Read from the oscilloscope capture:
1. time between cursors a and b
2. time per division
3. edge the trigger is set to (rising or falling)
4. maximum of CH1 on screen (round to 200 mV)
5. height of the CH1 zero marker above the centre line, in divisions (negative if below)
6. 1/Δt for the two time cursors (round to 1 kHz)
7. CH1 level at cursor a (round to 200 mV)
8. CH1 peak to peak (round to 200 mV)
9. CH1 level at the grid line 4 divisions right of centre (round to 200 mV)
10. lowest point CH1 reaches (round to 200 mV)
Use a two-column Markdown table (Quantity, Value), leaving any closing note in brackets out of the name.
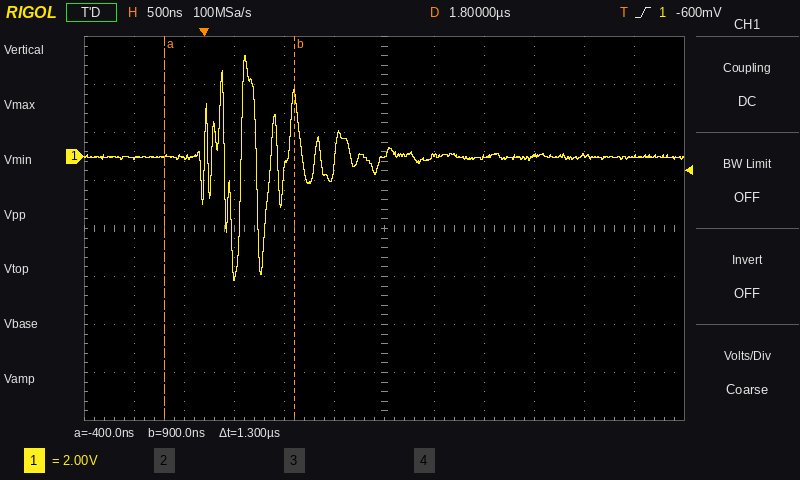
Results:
| Quantity | Value |
|---|---|
| time between cursors a and b | 1.3 µs |
| time per division | 500 ns |
| edge the trigger is set to | rising |
| maximum of CH1 on screen | 4.2 V |
| height of the CH1 zero marker above the centre line, in divisions | +1.5 div |
| 1/Δt for the two time cursors | 769 kHz |
| CH1 level at cursor a | 0.0 V |
| CH1 peak to peak | 9.4 V |
| CH1 level at the grid line 4 divisions right of centre | 0.0 V |
| lowest point CH1 reaches | -5.2 V |
